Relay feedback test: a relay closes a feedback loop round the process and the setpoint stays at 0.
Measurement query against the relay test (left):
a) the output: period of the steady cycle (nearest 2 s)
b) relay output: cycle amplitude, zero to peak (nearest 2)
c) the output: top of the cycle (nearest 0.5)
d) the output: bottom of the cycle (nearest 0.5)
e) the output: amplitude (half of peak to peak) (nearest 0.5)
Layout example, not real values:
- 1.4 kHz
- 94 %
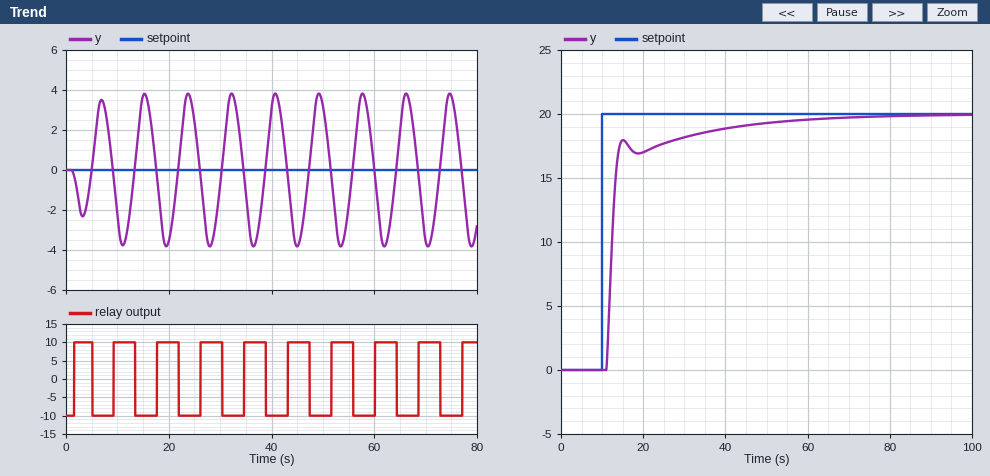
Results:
- 8 s
- 10
- 4.0
- -4.0
- 4.0
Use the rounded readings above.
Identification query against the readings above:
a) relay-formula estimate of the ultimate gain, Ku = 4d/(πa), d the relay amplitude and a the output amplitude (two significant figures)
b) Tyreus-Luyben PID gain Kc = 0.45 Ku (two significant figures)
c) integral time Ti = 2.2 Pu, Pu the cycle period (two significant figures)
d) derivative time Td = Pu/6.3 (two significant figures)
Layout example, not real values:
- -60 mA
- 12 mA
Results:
- 3.2
- 1.4
- 18 s
- 1.3 s
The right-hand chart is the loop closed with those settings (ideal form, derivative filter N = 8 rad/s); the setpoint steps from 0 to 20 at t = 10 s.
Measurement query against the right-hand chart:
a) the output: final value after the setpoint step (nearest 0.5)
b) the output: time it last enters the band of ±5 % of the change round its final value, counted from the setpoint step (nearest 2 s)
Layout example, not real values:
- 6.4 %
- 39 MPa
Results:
- 20.0
- 32 s
